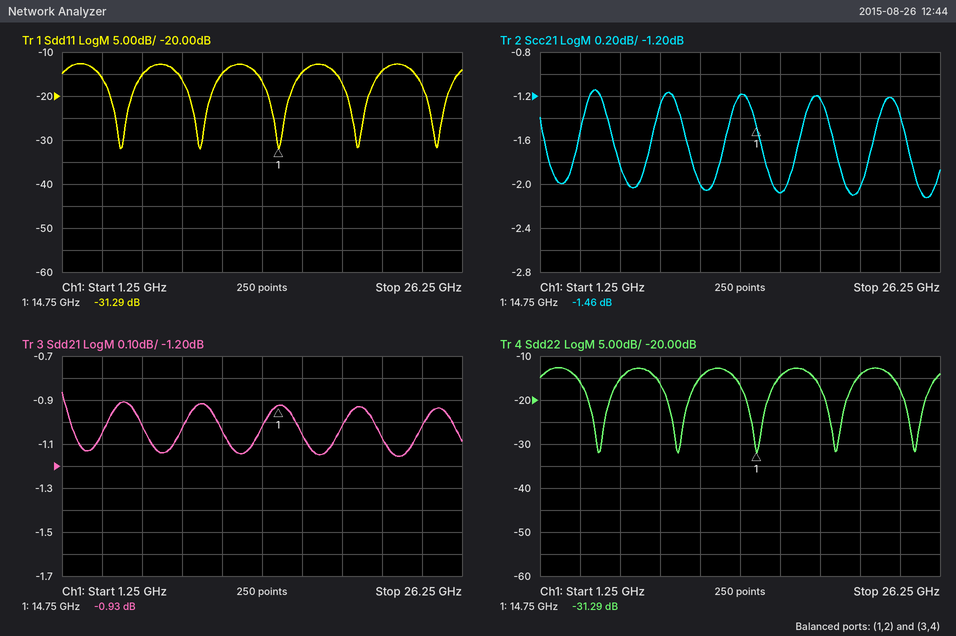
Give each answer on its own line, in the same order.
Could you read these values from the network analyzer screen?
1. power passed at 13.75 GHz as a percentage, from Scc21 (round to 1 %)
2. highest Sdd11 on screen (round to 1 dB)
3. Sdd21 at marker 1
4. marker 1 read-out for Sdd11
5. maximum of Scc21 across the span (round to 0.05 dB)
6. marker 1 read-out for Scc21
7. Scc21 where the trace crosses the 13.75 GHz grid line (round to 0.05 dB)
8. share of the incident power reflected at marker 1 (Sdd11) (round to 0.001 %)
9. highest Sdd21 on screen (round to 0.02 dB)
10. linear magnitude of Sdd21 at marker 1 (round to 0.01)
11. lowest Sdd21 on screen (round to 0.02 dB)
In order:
76 %
-13 dB
-0.93 dB
-31.29 dB
-1.15 dB
-1.46 dB
-1.20 dB
0.074 %
-0.86 dB
0.90
-1.16 dB
